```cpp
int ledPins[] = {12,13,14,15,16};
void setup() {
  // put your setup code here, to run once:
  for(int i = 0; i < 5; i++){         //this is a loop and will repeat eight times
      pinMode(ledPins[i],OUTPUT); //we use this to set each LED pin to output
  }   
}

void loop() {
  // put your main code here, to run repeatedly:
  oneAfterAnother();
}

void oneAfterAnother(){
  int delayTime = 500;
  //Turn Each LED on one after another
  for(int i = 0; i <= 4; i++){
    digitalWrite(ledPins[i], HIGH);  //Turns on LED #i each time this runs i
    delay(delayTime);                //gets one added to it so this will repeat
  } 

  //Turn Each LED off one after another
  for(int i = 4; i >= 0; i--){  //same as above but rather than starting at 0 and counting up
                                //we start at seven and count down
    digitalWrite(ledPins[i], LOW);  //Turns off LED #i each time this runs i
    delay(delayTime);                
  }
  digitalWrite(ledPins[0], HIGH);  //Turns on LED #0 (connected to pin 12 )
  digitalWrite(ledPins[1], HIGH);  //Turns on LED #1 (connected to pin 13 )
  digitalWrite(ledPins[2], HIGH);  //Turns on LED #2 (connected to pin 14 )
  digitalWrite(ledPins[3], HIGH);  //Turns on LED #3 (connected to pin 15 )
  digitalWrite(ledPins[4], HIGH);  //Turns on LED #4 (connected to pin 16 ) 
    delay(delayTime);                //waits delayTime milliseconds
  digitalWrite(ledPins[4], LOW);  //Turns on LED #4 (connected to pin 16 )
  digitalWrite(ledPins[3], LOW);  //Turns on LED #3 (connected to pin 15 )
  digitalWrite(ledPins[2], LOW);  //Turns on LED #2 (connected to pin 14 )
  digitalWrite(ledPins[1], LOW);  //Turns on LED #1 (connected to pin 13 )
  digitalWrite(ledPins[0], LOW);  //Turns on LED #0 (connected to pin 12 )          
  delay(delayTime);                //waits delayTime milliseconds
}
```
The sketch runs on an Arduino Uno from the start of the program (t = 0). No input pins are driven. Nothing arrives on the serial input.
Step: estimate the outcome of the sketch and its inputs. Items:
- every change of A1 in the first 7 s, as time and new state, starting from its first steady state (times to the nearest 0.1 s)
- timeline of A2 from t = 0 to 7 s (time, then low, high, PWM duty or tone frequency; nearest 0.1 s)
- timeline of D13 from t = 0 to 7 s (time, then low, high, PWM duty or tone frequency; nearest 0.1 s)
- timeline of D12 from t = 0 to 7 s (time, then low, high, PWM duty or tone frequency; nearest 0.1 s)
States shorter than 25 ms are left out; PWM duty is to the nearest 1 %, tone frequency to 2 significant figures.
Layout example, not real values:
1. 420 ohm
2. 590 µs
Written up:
1. 0 s low; 1.5 s high; 3 s low; 5 s high; 5.5 s low
2. 0 s low; 2 s high; 2.5 s low; 5 s high; 5.5 s low
3. 0 s low; 0.5 s high; 4 s low; 5 s high; 5.5 s low; 6.5 s high
4. 0 s high; 4.5 s low; 5 s high; 5.5 s low; 6 s high
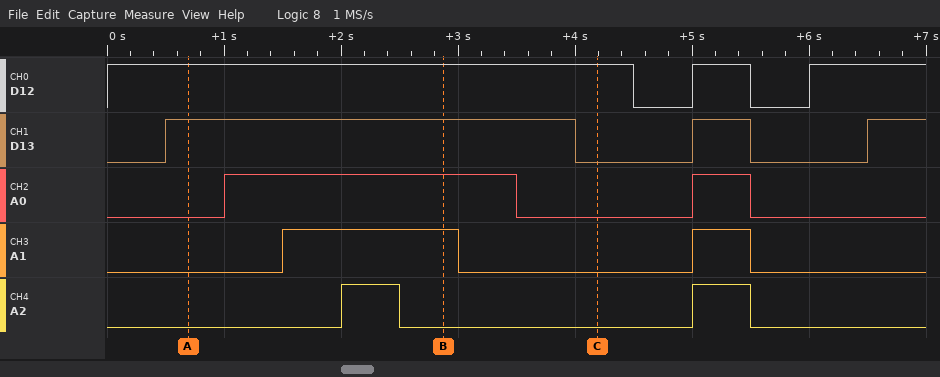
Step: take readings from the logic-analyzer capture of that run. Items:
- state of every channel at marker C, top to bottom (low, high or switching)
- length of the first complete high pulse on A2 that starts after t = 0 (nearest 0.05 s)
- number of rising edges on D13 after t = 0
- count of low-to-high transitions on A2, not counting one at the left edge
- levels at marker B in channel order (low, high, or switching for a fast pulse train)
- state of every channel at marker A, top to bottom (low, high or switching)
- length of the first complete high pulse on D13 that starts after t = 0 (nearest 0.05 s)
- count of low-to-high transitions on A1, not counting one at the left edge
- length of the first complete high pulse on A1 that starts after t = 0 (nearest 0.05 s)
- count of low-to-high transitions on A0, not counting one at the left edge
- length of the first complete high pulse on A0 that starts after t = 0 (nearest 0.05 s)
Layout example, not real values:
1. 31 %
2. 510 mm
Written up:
1. D12 high, D13 low, A0 low, A1 low, A2 low
2. 0.50 s
3. 3
4. 2
5. D12 high, D13 high, A0 high, A1 high, A2 low
6. D12 high, D13 high, A0 low, A1 low, A2 low
7. 3.50 s
8. 2
9. 1.50 s
10. 2
11. 2.50 s
